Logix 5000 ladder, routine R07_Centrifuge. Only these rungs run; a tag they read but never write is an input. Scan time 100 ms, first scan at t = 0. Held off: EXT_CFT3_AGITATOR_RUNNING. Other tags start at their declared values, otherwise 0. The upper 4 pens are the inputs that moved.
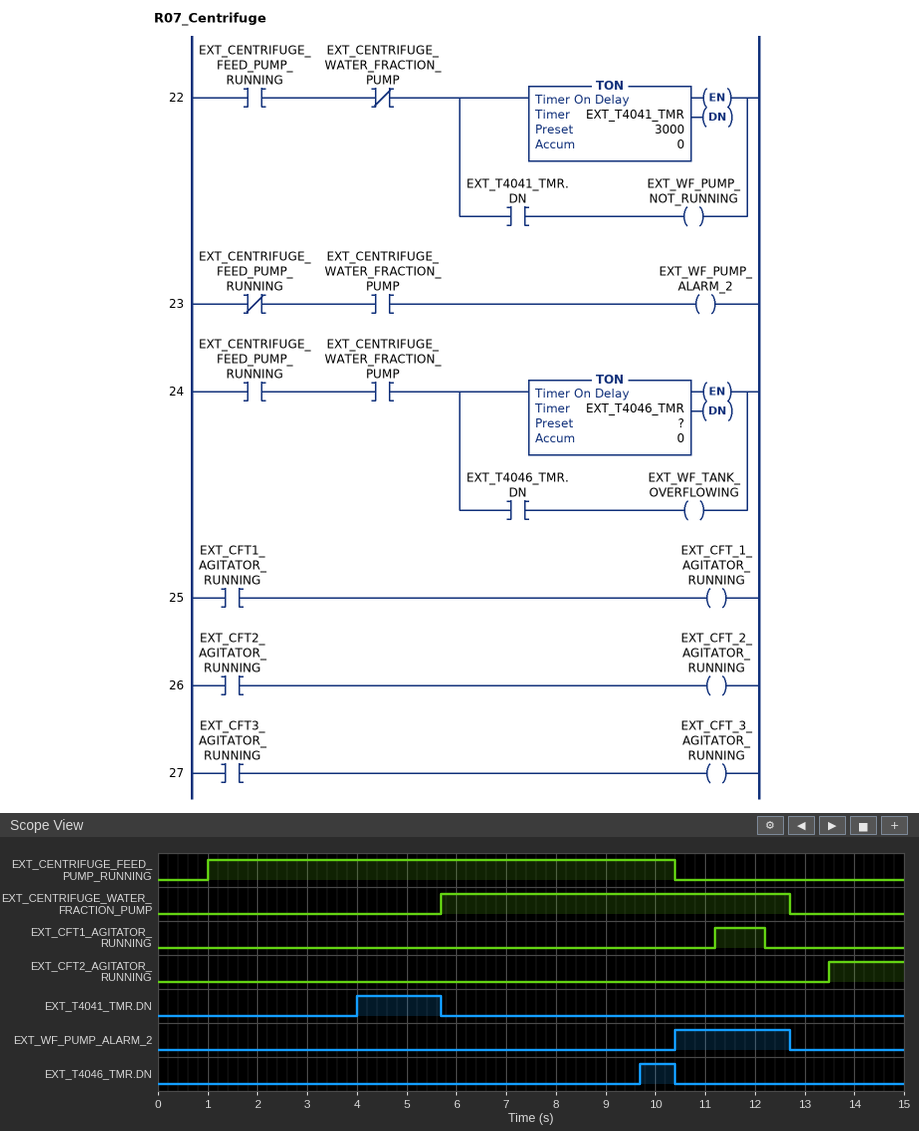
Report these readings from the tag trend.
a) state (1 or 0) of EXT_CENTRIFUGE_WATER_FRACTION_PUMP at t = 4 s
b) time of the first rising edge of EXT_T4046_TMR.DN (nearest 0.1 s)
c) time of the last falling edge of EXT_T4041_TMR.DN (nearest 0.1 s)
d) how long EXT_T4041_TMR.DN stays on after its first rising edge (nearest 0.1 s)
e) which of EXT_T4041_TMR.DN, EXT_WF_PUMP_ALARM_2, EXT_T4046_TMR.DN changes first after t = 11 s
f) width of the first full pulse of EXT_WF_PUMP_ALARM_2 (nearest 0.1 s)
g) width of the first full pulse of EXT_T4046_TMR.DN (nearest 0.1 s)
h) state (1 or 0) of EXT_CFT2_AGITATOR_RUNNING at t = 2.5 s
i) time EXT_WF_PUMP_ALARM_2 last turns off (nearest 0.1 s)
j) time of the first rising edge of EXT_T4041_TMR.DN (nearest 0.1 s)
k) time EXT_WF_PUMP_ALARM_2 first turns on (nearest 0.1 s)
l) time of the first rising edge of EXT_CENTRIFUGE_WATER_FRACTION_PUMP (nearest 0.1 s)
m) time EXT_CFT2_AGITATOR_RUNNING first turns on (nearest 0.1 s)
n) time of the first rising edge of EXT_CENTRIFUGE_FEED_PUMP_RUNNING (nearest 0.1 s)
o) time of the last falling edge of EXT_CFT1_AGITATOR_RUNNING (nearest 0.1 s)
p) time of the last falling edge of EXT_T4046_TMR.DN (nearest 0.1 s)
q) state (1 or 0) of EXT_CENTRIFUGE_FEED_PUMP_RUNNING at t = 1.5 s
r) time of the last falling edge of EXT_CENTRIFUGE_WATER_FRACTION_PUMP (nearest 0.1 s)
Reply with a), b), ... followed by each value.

a) 0
b) 9.7 s
c) 5.7 s
d) 1.7 s
e) EXT_WF_PUMP_ALARM_2
f) 2.3 s
g) 0.7 s
h) 0
i) 12.7 s
j) 4.0 s
k) 10.4 s
l) 5.7 s
m) 13.5 s
n) 1.0 s
o) 12.2 s
p) 10.4 s
q) 1
r) 12.7 s
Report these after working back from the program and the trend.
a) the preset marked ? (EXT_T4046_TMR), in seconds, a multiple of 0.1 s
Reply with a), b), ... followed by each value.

a) 4.0 s
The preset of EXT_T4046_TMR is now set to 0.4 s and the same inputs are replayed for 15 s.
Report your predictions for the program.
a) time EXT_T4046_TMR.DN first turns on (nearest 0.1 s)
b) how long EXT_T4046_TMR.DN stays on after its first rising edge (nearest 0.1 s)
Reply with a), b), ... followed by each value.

a) 6.1 s
b) 4.3 s
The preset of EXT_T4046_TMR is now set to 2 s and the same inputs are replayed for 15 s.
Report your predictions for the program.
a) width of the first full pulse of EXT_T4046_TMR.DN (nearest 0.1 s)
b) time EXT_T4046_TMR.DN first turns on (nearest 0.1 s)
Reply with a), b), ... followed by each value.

a) 2.7 s
b) 7.7 s
